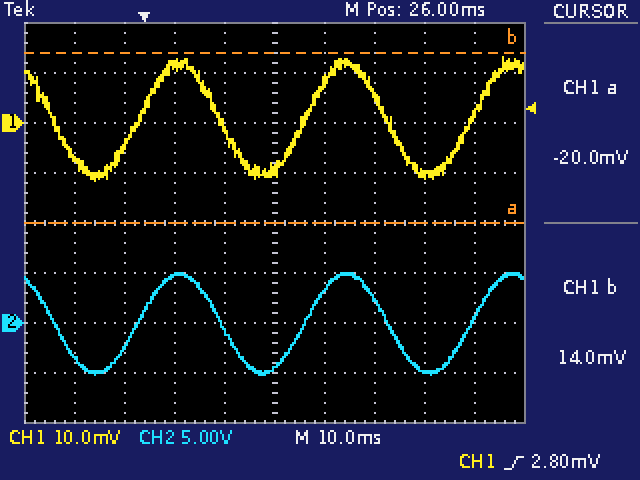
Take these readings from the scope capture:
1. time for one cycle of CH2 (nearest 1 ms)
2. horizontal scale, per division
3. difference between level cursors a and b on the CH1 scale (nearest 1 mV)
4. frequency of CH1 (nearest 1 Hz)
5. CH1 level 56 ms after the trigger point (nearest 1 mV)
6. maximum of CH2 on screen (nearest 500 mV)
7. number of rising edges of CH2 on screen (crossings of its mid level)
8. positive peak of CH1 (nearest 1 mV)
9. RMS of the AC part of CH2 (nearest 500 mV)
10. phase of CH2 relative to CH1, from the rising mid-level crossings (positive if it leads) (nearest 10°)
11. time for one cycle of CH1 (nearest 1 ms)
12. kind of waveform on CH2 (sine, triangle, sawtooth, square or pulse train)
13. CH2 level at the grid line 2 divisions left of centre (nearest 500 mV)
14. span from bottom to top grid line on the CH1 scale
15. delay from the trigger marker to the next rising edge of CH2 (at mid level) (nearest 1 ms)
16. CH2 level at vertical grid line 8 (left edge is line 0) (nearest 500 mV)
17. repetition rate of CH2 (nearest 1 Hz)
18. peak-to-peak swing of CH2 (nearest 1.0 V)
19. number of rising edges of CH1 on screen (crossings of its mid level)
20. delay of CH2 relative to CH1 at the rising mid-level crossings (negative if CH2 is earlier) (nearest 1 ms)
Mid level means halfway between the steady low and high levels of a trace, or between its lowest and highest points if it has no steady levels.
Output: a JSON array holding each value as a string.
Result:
["33 ms", "10 ms", "34 mV", "30 Hz", "-10 mV", "5.0 V", "3", "13 mV", "3.5 V", "0°", "33 ms", "sine", "4.5 V", "80 mV", "32 ms", "-5.0 V", "30 Hz", "10.0 V", "3", "0 ms"]
